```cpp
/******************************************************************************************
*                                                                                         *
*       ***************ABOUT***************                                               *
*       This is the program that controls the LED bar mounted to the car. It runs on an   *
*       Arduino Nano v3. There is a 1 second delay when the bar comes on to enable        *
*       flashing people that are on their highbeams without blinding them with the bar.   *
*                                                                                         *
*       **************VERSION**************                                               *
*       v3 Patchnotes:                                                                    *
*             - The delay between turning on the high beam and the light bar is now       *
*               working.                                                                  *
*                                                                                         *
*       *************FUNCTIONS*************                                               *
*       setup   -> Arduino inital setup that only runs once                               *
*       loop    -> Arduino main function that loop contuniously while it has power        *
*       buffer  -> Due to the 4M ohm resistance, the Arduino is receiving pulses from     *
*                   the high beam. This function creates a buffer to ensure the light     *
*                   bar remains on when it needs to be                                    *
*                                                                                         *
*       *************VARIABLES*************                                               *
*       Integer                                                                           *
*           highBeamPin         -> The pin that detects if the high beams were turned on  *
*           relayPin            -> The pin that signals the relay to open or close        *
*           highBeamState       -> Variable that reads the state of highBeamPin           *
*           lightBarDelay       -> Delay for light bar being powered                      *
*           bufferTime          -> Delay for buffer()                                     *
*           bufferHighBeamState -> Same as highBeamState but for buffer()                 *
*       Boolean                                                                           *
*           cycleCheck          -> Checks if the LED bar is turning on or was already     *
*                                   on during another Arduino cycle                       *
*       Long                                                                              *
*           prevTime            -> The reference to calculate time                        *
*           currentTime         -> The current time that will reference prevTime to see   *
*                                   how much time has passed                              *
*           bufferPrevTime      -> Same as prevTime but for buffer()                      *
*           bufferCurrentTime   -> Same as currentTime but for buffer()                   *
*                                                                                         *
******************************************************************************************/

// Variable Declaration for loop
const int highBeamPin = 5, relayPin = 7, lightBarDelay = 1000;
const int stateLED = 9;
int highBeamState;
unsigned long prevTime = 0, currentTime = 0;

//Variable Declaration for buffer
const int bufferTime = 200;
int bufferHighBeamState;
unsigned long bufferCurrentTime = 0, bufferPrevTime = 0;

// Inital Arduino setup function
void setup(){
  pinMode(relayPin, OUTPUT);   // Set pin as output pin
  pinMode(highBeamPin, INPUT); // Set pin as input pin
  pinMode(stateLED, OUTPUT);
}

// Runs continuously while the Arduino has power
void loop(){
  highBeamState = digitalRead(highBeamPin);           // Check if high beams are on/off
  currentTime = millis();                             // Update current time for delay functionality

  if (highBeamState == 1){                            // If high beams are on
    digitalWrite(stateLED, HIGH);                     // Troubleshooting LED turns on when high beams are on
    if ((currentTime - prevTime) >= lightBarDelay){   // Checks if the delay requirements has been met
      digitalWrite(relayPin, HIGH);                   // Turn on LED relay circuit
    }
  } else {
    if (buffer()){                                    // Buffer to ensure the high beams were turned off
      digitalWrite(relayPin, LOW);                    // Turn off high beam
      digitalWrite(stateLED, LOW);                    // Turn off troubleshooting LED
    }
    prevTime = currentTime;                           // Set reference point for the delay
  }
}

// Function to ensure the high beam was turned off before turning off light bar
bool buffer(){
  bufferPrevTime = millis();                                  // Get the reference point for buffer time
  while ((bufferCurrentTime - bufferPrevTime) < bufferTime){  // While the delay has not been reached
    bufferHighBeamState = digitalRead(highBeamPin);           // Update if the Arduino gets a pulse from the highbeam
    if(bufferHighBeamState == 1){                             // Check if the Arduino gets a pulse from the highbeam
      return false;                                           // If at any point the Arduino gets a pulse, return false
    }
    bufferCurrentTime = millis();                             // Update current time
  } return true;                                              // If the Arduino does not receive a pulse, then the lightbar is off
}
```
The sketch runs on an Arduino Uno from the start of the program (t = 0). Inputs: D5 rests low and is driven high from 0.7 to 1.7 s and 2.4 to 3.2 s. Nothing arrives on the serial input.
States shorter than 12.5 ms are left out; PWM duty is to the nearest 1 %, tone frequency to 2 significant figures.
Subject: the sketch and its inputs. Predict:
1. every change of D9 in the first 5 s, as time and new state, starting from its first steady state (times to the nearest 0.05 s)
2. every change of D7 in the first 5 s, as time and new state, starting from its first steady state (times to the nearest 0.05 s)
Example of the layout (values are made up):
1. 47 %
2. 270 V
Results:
1. 0 s low; 0.7 s high; 1.7 s low; 2.4 s high; 3.2 s low
2. 0 s low; 1.6 s high; 1.7 s low
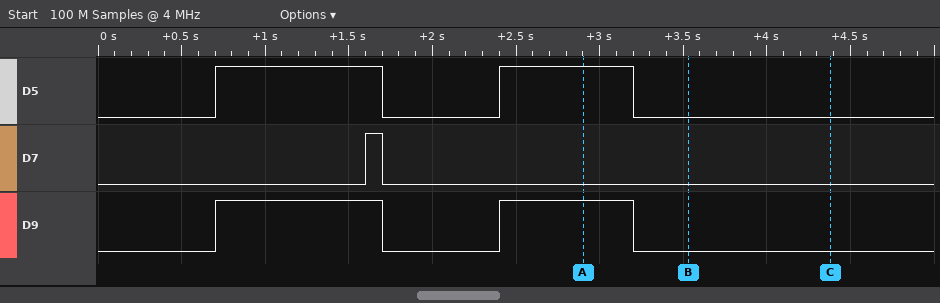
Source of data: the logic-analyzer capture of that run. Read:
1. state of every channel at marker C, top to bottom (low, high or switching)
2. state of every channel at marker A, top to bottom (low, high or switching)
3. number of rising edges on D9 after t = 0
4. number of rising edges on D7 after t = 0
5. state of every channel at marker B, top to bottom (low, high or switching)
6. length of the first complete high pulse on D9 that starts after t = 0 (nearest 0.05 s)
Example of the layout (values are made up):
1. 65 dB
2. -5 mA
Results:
1. D5 low, D7 low, D9 low
2. D5 high, D7 low, D9 high
3. 2
4. 1
5. D5 low, D7 low, D9 low
6. 1.00 s
